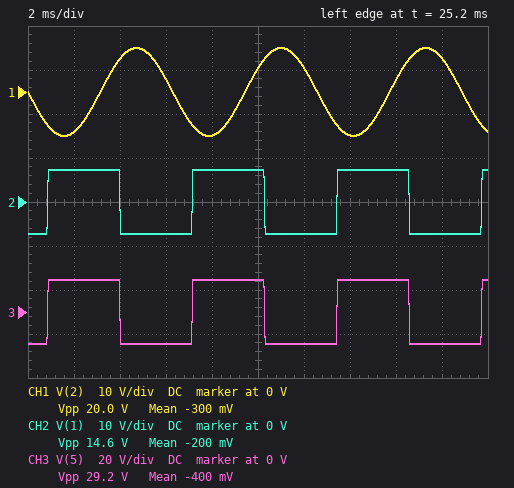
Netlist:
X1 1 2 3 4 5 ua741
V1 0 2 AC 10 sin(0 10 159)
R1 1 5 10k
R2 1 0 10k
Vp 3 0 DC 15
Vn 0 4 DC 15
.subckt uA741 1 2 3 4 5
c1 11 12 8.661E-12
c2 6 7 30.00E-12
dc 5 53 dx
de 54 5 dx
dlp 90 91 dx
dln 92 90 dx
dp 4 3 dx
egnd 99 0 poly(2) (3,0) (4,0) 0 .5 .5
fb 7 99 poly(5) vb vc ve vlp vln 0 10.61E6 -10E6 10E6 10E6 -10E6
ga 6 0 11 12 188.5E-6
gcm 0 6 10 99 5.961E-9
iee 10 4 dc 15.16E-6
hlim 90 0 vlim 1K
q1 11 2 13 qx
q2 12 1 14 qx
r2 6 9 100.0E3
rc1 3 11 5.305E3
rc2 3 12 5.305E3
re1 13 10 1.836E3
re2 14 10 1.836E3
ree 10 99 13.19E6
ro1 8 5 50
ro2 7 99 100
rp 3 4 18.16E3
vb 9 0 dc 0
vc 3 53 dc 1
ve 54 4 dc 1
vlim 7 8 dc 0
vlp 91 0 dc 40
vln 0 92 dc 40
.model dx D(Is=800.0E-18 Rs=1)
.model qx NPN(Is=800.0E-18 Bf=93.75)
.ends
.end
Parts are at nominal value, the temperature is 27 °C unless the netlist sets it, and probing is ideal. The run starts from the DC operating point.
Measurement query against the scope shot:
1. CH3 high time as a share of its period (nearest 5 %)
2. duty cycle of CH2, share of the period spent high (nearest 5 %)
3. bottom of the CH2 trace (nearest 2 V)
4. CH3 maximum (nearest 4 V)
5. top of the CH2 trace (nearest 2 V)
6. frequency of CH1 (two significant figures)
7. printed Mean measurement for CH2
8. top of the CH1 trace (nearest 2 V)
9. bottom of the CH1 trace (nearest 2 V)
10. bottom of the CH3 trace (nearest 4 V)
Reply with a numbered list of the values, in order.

1. 50 %
2. 50 %
3. -8 V
4. 16 V
5. 8 V
6. 160 Hz
7. -200 mV
8. 10 V
9. -10 V
10. -16 V
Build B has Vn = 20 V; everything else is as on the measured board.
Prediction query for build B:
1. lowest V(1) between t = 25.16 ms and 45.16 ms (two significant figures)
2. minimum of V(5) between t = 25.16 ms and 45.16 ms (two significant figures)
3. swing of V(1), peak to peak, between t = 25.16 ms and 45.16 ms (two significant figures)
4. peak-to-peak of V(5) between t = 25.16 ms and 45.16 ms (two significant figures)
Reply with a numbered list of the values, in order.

1. -9.8 V
2. -20 V
3. 17 V
4. 34 V
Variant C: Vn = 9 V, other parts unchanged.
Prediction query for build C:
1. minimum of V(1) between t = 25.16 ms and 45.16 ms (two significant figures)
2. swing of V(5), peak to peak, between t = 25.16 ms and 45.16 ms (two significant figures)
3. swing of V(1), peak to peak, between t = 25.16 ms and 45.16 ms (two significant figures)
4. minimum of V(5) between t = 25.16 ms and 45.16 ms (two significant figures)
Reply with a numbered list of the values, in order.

1. -4.3 V
2. 23 V
3. 12 V
4. -8.6 V
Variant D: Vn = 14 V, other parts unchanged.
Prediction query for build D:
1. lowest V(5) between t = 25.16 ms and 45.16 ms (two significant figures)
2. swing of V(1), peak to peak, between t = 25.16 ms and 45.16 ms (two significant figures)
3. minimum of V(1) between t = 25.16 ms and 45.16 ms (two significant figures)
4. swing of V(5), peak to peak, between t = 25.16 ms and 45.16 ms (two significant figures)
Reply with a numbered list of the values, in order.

1. -14 V
2. 14 V
3. -6.8 V
4. 28 V
